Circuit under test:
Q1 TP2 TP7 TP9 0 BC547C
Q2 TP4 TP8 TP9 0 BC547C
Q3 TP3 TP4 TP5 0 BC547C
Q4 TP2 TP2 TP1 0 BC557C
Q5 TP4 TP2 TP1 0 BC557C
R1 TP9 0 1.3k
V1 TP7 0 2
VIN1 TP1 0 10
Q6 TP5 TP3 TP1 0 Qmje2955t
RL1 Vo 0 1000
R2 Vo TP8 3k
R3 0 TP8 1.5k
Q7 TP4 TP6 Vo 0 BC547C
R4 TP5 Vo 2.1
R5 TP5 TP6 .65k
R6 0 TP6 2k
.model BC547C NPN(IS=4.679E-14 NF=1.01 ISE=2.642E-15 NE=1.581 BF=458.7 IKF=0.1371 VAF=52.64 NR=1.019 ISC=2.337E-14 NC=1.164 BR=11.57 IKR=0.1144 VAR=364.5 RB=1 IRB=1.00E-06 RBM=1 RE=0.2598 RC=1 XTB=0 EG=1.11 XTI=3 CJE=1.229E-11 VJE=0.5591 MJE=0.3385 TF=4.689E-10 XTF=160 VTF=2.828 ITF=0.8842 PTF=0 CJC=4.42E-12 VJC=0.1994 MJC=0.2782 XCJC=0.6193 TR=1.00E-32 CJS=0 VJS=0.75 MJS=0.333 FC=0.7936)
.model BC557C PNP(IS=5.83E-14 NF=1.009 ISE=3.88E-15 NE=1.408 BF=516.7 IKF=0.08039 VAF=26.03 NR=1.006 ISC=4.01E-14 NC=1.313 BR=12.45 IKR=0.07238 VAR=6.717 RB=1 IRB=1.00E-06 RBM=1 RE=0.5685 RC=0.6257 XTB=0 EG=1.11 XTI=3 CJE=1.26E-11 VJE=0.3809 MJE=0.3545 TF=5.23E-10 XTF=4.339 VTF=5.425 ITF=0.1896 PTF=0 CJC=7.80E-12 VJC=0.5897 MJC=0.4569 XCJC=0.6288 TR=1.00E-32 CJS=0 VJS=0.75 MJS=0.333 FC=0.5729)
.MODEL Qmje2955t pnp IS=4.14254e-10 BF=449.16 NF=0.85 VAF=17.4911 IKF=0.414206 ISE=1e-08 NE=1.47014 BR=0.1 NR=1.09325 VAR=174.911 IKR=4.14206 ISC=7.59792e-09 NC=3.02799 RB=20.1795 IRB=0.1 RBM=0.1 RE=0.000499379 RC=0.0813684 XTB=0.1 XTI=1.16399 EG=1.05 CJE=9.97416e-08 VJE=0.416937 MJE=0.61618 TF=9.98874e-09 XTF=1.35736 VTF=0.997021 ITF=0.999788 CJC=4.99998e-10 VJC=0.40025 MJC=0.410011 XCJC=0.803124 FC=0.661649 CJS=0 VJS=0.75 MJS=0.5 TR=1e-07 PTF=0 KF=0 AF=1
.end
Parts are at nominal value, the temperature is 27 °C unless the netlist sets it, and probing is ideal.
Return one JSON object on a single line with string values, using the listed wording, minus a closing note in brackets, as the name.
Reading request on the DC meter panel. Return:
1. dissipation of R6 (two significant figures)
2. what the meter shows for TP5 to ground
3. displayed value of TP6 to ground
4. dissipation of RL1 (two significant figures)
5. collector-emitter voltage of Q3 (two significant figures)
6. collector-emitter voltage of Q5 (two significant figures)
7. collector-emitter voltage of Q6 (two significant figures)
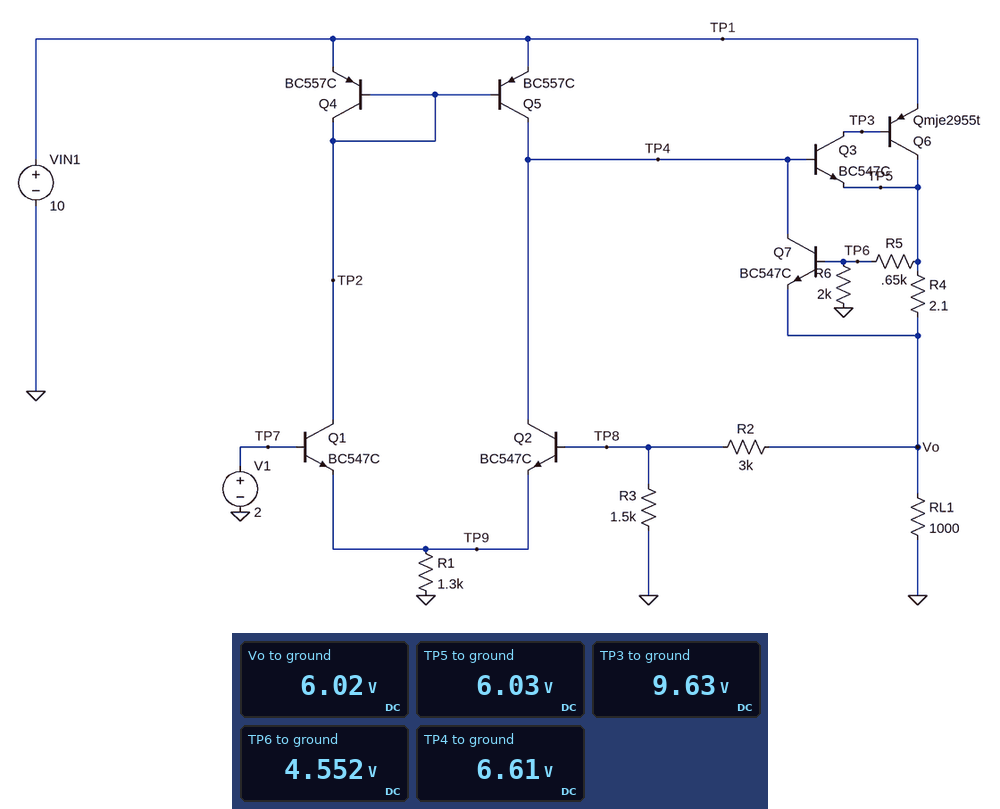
{"dissipation of R6": "10 mW", "what the meter shows for TP5 to ground": "6.03 V", "displayed value of TP6 to ground": "4.552 V", "dissipation of RL1": "36 mW", "collector-emitter voltage of Q3": "3.6 V", "collector-emitter voltage of Q5": "-3.4 V", "collector-emitter voltage of Q6": "-4.0 V"}
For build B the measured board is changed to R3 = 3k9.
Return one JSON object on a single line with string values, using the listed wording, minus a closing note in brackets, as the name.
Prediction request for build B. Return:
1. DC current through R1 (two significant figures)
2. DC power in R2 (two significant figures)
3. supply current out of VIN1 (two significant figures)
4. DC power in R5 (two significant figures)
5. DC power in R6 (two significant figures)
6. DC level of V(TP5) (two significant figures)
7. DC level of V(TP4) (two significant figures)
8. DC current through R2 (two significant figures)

{"DC current through R1": "1.1 mA", "DC power in R2": "800 µW", "supply current out of VIN1": "6.5 mA", "DC power in R5": "1.2 mW", "DC power in R6": "3.6 mW", "DC level of V(TP5)": "3.6 V", "DC level of V(TP4)": "4.1 V", "DC current through R2": "520 µA"}
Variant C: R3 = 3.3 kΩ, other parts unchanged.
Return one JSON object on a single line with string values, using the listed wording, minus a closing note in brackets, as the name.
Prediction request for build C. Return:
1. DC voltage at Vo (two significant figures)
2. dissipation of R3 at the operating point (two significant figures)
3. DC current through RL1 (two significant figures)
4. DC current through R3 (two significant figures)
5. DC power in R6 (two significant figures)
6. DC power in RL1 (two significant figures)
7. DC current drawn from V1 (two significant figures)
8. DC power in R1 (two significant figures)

{"DC voltage at Vo": "3.8 V", "dissipation of R3 at the operating point": "1.2 mW", "DC current through RL1": "3.8 mA", "DC current through R3": "610 µA", "DC power in R6": "4.2 mW", "DC power in RL1": "15 mW", "DC current drawn from V1": "940 nA", "DC power in R1": "1.5 mW"}
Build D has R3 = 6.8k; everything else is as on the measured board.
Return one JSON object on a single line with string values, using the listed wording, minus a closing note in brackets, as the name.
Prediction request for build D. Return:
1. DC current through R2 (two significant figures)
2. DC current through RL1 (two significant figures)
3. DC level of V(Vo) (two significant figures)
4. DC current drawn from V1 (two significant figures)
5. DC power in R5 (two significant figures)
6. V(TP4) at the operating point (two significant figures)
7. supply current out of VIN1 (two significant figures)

{"DC current through R2": "300 µA", "DC current through RL1": "2.9 mA", "DC level of V(Vo)": "2.9 V", "DC current drawn from V1": "930 nA", "DC power in R5": "780 µW", "V(TP4) at the operating point": "3.5 V", "supply current out of VIN1": "5.4 mA"}
